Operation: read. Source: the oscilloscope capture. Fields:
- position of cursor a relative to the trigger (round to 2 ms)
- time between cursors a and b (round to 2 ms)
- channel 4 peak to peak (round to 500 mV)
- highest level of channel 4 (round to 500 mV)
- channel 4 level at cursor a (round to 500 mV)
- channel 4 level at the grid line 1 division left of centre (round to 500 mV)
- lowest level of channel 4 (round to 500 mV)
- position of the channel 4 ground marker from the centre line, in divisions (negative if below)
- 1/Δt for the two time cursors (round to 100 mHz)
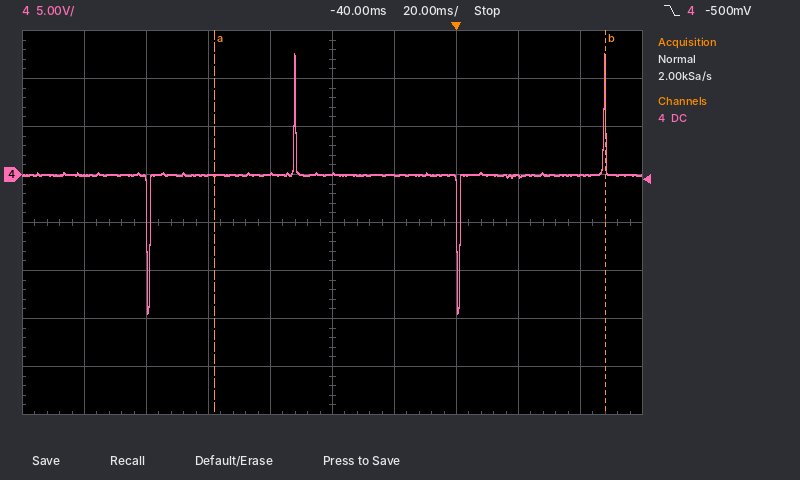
-78 ms
126 ms
27.0 V
12.5 V
0.0 V
0.0 V
-14.5 V
+1.0 div
7.9 Hz
